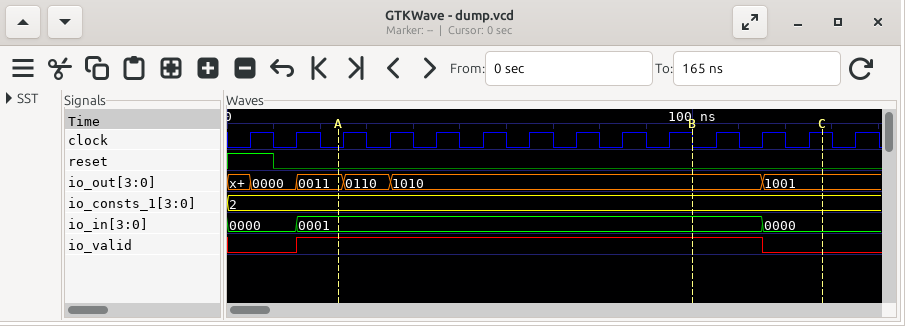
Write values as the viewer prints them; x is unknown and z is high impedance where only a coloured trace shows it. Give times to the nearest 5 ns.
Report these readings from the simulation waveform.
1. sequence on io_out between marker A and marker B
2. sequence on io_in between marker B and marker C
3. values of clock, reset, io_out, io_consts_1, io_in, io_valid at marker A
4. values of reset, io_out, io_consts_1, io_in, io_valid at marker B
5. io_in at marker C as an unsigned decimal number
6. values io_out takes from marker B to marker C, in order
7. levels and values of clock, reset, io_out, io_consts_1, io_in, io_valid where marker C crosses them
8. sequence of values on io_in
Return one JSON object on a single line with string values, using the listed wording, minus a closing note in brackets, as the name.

{"sequence on io_out between marker A and marker B": "0011, 0110, 1010", "sequence on io_in between marker B and marker C": "0001, 0000", "values of clock, reset, io_out, io_consts_1, io_in, io_valid at marker A": "clock=0, reset=0, io_out=0011, io_consts_1=2, io_in=0001, io_valid=1", "values of reset, io_out, io_consts_1, io_in, io_valid at marker B": "reset=0, io_out=1010, io_consts_1=2, io_in=0001, io_valid=1", "io_in at marker C as an unsigned decimal number": "0", "values io_out takes from marker B to marker C, in order": "1010, 1001", "levels and values of clock, reset, io_out, io_consts_1, io_in, io_valid where marker C crosses them": "clock=1, reset=0, io_out=1001, io_consts_1=2, io_in=0000, io_valid=0", "sequence of values on io_in": "0000, 0001, 0000"}
